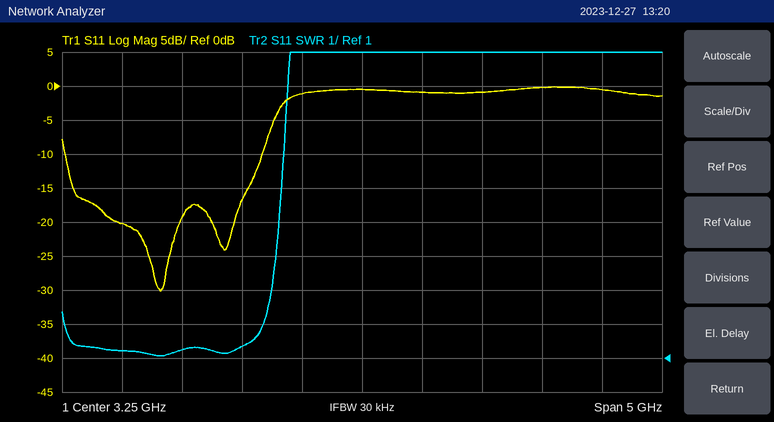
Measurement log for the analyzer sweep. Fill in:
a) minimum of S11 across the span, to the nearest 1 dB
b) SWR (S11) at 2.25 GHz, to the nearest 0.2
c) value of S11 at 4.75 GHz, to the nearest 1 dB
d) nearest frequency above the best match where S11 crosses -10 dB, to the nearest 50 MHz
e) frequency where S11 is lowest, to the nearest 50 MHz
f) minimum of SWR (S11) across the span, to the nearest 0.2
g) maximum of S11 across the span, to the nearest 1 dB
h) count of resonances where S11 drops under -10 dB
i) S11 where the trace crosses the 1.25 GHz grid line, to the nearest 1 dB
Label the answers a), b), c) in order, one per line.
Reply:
a) -30 dB
b) 1.4
c) 0 dB
d) 2.40 GHz
e) 1.55 GHz
f) 1.0
g) 0 dB
h) 2
i) -20 dB
